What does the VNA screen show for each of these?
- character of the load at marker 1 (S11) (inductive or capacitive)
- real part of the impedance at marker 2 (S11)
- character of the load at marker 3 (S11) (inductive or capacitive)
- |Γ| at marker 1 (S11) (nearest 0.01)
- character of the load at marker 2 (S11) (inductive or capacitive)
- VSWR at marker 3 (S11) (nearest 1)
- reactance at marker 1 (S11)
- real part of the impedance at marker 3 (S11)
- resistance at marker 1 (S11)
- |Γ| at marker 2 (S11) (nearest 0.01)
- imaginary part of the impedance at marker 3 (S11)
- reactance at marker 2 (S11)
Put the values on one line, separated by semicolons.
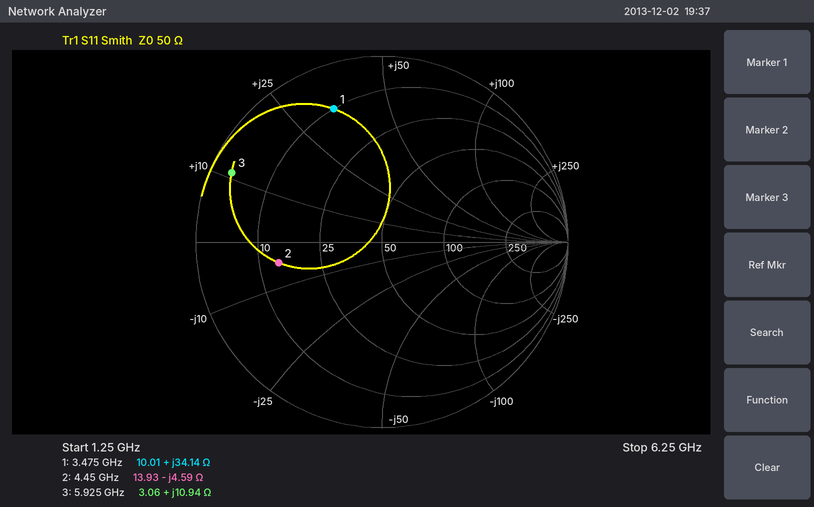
inductive; 13.93 Ω; inductive; 0.76; capacitive; 17; +34.14 Ω; 3.06 Ω; 10.01 Ω; 0.57; +10.94 Ω; -4.59 Ω
